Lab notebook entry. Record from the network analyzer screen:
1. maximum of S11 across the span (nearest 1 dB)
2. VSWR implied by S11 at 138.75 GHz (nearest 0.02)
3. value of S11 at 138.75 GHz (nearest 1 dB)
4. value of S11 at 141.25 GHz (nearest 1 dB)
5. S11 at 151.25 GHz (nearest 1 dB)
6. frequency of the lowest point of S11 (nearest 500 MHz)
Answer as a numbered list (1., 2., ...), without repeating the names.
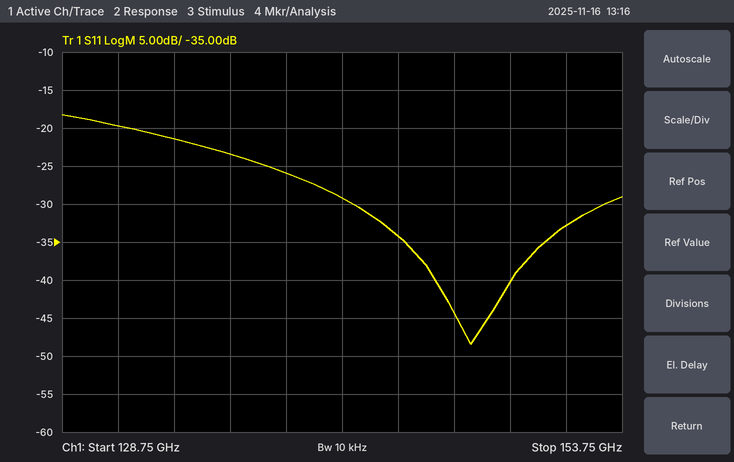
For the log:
1. -18 dB
2. 1.10
3. -26 dB
4. -29 dB
5. -33 dB
6. 147.0 GHz
